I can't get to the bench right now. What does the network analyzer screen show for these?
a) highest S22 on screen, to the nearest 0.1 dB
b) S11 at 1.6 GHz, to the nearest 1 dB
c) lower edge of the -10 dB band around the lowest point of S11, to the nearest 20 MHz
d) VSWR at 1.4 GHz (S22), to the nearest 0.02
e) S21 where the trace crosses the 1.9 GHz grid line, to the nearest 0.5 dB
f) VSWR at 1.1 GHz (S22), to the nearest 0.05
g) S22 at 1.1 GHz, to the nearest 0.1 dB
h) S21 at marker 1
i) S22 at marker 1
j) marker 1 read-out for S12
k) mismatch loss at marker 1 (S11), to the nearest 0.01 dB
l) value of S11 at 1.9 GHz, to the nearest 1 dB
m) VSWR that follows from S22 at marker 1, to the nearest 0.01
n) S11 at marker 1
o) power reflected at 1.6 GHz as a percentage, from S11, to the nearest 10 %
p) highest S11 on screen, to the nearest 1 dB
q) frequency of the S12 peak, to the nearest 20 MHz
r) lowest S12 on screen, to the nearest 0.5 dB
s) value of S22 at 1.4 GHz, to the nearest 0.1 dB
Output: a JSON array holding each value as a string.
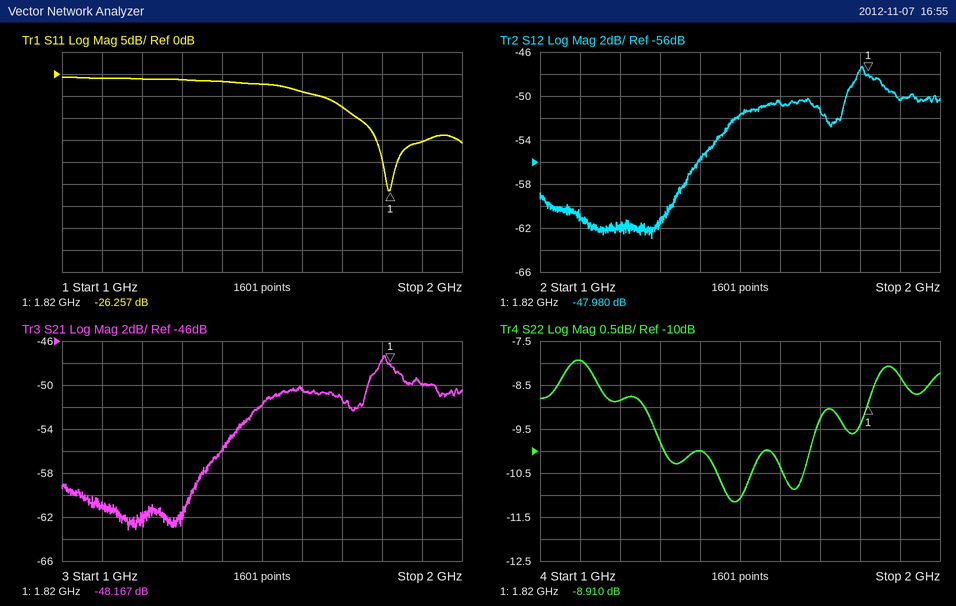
["-7.9 dB", "-4 dB", "1.74 GHz", "1.92", "-50.0 dB", "2.35", "-7.9 dB", "-48.167 dB", "-8.910 dB", "-47.980 dB", "0.01 dB", "-15 dB", "2.12", "-26.257 dB", "40 %", "-1 dB", "1.80 GHz", "-63.0 dB", "-10.0 dB"]
